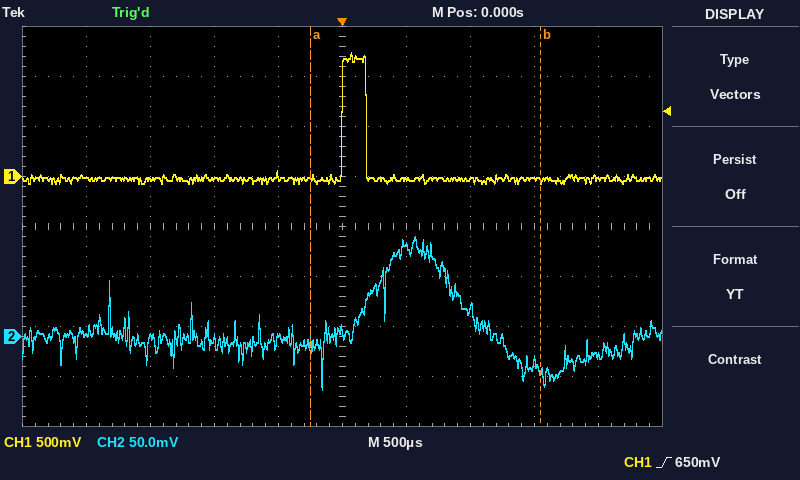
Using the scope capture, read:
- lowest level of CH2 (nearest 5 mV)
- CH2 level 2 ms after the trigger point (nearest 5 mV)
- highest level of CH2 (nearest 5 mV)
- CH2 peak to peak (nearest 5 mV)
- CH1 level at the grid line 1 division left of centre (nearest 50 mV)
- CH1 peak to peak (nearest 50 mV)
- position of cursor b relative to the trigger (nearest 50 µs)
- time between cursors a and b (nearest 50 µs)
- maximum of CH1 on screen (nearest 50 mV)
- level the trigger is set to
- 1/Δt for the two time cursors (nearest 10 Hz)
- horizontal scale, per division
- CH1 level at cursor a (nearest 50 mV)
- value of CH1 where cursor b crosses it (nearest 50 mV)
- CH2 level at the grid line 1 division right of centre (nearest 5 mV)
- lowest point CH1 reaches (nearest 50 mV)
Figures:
-55 mV
-20 mV
100 mV
155 mV
0 mV
1.30 V
+1.55 ms
1.80 ms
1.25 V
650 mV
560 Hz
500 µs
0 mV
-50 mV
90 mV
-50 mV
